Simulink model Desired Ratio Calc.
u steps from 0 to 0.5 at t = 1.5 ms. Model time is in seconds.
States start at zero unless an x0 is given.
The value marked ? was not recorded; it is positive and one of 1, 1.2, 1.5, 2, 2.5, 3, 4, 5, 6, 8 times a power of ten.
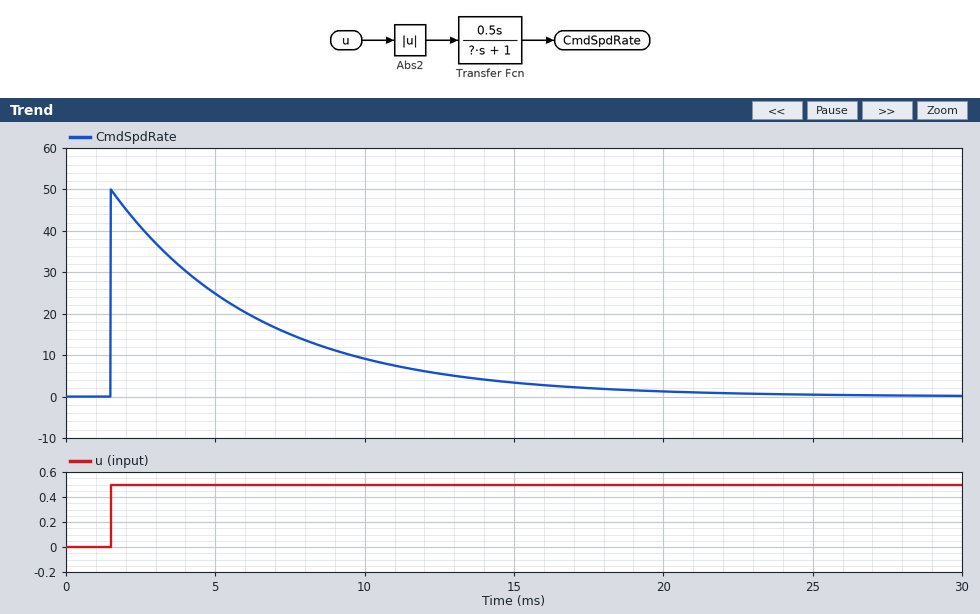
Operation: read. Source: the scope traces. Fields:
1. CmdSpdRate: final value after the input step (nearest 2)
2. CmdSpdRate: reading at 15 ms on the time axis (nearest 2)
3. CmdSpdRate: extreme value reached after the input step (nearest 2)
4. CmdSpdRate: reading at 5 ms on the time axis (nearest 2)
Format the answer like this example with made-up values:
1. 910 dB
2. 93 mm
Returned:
1. 0
2. 4
3. 50
4. 24
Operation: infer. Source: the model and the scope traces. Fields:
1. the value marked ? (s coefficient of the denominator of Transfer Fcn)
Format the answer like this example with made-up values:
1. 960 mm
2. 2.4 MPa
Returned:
1. 0.005
